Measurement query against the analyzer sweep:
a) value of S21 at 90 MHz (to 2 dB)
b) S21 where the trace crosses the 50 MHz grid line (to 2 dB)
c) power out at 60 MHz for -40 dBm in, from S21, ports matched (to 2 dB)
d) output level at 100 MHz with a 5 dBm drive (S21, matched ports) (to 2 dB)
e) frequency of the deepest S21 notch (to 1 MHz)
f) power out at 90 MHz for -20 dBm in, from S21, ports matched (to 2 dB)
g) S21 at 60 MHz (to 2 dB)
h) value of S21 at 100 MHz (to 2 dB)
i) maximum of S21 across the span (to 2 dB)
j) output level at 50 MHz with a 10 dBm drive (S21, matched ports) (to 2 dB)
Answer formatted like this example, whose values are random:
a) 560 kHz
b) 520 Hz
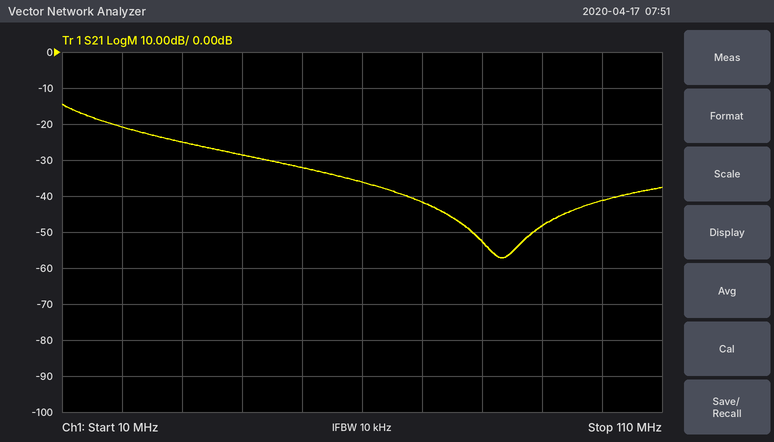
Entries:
a) -48 dB
b) -32 dB
c) -76 dBm
d) -36 dBm
e) 83 MHz
f) -68 dBm
g) -36 dB
h) -42 dB
i) -14 dB
j) -22 dBm
